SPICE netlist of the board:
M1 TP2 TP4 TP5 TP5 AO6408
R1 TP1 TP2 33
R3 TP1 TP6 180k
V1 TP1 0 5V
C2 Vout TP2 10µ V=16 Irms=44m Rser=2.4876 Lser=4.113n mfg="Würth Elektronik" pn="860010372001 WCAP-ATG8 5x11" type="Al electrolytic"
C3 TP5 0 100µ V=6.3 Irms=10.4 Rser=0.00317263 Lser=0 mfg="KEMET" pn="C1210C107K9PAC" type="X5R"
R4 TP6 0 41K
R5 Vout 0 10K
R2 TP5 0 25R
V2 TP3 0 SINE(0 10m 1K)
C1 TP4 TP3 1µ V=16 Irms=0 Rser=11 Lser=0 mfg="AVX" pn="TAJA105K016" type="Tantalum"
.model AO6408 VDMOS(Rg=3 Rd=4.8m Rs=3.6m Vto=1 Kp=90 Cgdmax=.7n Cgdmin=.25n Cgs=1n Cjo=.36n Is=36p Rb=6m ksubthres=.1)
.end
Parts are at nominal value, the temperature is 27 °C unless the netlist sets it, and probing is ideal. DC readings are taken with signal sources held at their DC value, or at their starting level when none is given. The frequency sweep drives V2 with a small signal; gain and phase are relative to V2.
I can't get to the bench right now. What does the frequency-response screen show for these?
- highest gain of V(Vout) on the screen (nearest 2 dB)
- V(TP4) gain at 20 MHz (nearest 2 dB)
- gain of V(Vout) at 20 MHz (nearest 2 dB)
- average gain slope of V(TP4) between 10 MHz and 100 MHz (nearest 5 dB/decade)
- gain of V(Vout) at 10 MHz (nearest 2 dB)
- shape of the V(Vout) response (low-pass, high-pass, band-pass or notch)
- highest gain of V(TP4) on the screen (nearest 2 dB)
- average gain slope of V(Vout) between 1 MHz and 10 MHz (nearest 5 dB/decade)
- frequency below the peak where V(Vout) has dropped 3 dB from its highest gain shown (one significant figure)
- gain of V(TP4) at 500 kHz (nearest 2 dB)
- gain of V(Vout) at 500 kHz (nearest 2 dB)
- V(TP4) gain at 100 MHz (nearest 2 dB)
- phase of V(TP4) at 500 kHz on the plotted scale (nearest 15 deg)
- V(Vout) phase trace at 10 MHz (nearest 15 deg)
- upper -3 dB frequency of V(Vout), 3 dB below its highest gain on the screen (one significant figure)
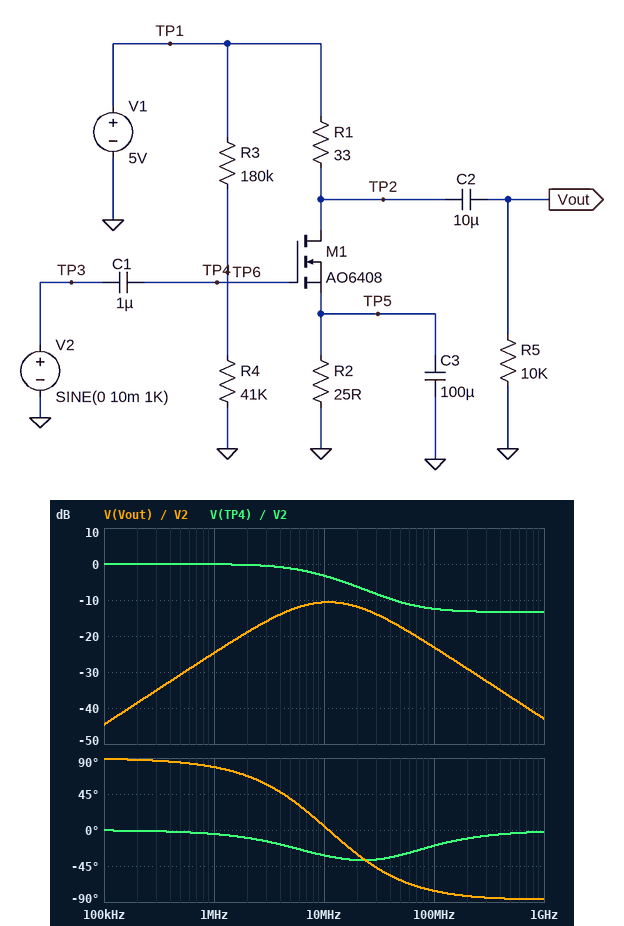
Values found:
-10 dB
-6 dB
-12 dB
-10 dB/decade
-10 dB
band-pass
0 dB
15 dB/decade
4 MHz
0 dB
-30 dB
-12 dB
0 deg
0 deg
30 MHz
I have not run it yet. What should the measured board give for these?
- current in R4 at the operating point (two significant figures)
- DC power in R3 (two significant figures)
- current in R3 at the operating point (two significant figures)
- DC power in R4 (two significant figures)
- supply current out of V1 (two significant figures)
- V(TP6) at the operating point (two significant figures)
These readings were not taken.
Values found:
23 µA
92 µW
23 µA
21 µW
23 µA
930 mV
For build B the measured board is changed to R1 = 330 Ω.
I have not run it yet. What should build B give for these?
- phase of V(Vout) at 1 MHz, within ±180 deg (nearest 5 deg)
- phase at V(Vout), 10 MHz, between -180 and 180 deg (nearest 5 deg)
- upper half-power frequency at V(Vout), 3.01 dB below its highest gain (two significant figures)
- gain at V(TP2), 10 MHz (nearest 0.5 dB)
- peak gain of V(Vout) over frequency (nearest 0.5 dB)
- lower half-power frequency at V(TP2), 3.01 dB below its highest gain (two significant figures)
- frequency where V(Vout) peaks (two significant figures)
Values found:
45 deg
-35 deg
13 MHz
-6.5 dB
-4.5 dB
970 kHz
3.5 MHz
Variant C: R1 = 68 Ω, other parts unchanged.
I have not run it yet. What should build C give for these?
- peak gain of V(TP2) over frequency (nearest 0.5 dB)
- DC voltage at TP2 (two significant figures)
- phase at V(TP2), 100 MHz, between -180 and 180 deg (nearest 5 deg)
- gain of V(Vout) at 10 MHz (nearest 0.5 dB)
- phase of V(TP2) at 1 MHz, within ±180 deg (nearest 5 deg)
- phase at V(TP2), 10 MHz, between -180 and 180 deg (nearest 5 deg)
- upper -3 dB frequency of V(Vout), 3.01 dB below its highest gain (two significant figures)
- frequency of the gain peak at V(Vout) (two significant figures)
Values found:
-7.5 dB
5.0 V
-80 deg
-8.0 dB
75 deg
-15 deg
20 MHz
7.7 MHz
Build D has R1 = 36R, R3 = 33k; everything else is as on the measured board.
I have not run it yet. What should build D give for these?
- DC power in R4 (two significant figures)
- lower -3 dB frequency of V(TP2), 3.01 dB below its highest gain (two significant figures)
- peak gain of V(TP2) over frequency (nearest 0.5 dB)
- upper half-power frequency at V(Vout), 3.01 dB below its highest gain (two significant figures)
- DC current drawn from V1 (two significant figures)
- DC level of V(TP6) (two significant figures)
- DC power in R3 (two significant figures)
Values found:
190 µW
4.1 MHz
-10.0 dB
27 MHz
68 µA
2.8 V
150 µW
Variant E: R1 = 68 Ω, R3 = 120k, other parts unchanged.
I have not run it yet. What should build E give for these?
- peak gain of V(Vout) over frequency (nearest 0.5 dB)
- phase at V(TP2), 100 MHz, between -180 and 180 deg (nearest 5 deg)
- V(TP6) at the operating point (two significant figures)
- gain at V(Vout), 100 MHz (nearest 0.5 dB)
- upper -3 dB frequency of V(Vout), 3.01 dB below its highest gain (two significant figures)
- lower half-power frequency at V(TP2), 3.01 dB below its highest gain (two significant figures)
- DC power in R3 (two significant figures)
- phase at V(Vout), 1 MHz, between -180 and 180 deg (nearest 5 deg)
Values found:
-7.5 dB
-80 deg
1.3 V
-23.0 dB
20 MHz
2.9 MHz
120 µW
75 deg
